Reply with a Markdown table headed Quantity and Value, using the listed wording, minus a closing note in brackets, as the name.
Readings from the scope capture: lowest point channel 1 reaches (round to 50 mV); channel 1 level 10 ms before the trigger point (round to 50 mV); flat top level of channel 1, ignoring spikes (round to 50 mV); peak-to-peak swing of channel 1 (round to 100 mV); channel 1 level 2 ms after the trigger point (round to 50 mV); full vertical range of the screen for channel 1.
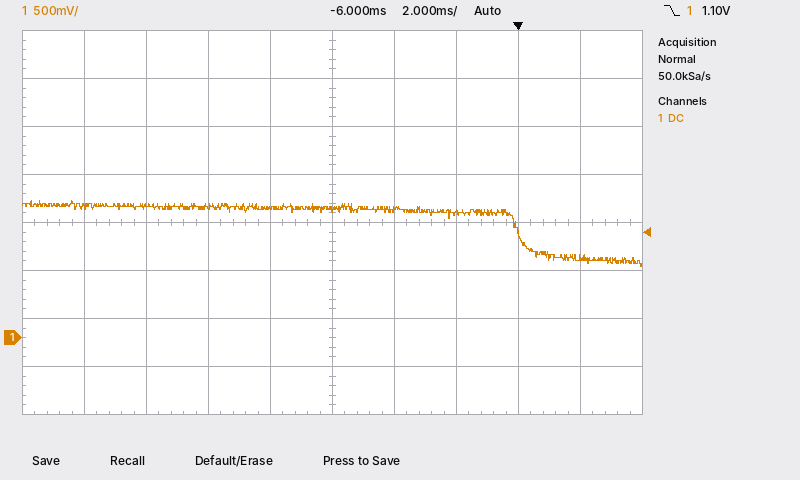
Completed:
| Quantity | Value |
|---|---|
| lowest point channel 1 reaches | 750 mV |
| channel 1 level 10 ms before the trigger point | 1.35 V |
| flat top level of channel 1, ignoring spikes | 1.35 V |
| peak-to-peak swing of channel 1 | 700 mV |
| channel 1 level 2 ms after the trigger point | 850 mV |
| full vertical range of the screen for channel 1 | 4 V |
